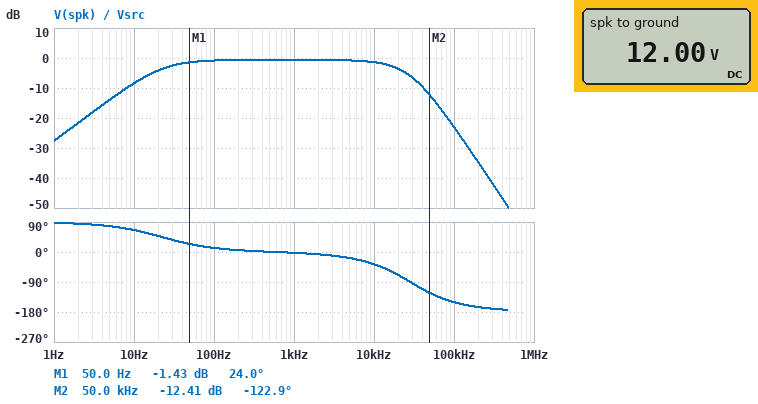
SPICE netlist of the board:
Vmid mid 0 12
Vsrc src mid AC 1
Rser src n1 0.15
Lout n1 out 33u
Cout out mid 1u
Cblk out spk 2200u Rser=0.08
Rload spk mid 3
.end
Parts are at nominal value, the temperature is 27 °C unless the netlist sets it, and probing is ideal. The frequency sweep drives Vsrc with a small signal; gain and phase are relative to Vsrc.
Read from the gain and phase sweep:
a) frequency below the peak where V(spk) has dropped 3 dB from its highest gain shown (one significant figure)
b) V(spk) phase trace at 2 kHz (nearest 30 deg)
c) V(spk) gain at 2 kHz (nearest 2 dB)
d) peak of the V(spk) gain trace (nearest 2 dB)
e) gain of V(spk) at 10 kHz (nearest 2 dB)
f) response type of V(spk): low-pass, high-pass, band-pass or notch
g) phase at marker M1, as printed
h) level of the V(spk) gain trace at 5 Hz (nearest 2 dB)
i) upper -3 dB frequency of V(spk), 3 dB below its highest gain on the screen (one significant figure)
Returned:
20 Hz
0 deg
0 dB
0 dB
-2 dB
band-pass
24.0 deg
-14 dB
20 kHz
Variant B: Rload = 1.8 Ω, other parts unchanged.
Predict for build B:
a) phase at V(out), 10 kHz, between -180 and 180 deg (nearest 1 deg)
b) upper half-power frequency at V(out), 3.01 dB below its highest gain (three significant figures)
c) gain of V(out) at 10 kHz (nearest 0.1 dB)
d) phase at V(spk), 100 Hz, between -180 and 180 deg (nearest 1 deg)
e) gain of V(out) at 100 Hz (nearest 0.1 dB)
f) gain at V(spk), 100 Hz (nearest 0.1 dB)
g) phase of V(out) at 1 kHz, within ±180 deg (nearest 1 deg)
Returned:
-50 deg
9.31 kHz
-3.3 dB
19 deg
-0.6 dB
-1.5 dB
-6 deg
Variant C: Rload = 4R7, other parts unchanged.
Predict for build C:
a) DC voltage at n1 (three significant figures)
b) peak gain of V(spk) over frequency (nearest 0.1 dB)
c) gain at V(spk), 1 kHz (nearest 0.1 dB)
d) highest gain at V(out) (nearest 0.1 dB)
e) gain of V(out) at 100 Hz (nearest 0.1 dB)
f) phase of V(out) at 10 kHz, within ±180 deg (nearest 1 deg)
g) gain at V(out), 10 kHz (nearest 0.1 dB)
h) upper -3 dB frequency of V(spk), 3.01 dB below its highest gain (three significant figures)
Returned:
12.0 V
-0.1 dB
-0.4 dB
0.1 dB
-0.3 dB
-26 deg
0 dB
31.2 kHz
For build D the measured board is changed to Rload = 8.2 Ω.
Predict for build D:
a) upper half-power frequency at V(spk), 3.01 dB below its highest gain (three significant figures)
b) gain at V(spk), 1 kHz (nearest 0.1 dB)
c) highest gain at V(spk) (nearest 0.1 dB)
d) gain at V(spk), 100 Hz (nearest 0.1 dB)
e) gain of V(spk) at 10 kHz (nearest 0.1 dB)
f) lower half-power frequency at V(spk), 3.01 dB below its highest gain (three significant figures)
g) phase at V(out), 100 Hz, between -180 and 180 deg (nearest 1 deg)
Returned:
33.2 kHz
-0.2 dB
3.3 dB
-0.3 dB
0.6 dB
7.85 kHz
0 deg
